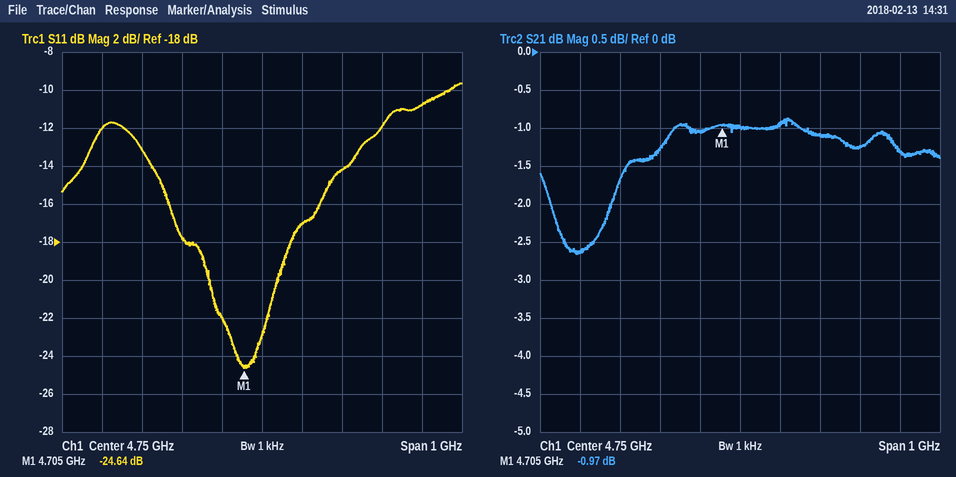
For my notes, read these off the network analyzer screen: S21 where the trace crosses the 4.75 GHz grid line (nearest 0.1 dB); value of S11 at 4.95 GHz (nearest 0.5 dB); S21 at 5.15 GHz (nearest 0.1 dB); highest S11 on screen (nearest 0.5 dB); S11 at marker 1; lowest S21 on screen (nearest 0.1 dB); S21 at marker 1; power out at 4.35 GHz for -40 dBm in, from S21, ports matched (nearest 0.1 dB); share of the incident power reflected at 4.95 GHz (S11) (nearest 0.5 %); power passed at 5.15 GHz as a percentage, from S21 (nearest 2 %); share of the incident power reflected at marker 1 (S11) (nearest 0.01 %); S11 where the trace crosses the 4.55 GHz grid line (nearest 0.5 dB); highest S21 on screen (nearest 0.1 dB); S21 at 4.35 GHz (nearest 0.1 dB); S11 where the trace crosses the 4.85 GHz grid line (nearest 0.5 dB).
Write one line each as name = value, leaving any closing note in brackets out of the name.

S21 where the trace crosses the 4.75 GHz grid line = -1.0 dB
value of S11 at 4.95 GHz = -14.0 dB
S21 at 5.15 GHz = -1.3 dB
highest S11 on screen = -9.5 dB
S11 at marker 1 = -24.64 dB
lowest S21 on screen = -2.7 dB
S21 at marker 1 = -0.97 dB
power out at 4.35 GHz for -40 dBm in, from S21, ports matched = -42.6 dBm
share of the incident power reflected at 4.95 GHz (S11) = 4.0 %
power passed at 5.15 GHz as a percentage, from S21 = 74 %
share of the incident power reflected at marker 1 (S11) = 0.34 %
S11 where the trace crosses the 4.55 GHz grid line = -18.0 dB
highest S21 on screen = -0.9 dB
S21 at 4.35 GHz = -2.6 dB
S11 where the trace crosses the 4.85 GHz grid line = -17.0 dB
